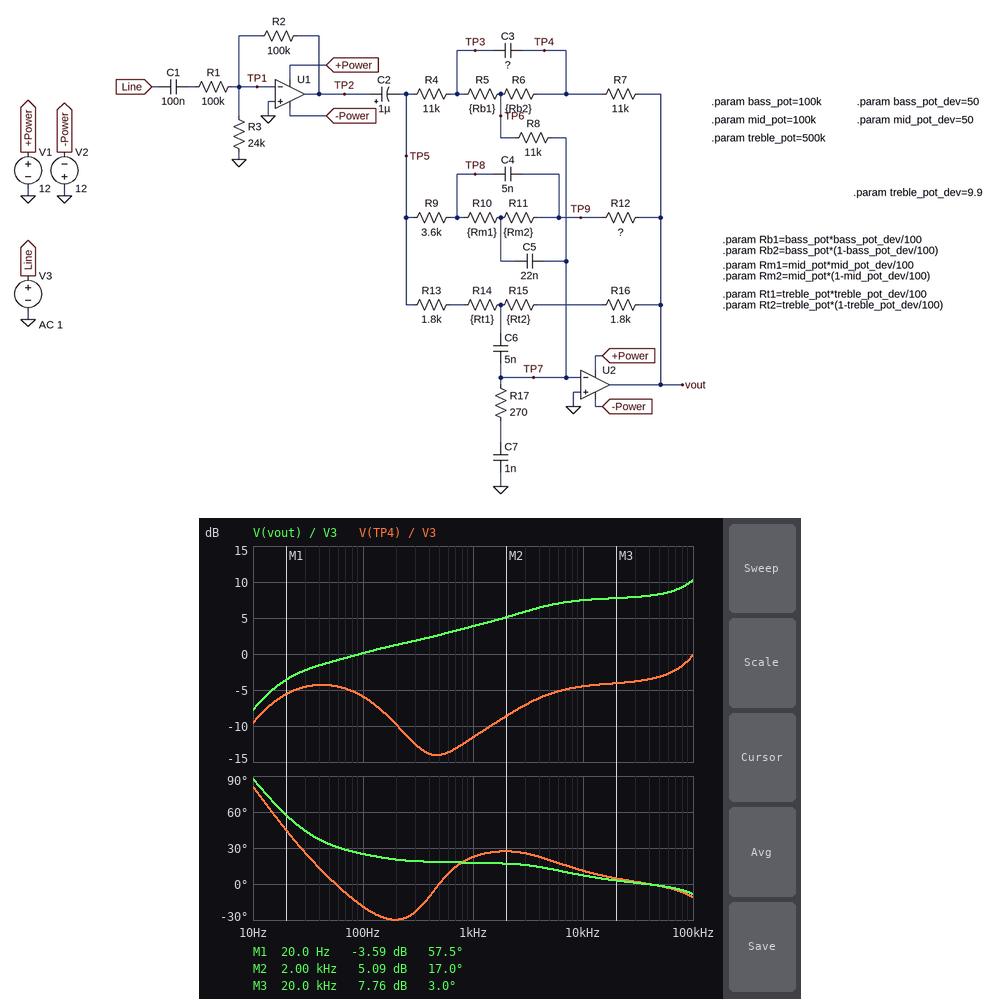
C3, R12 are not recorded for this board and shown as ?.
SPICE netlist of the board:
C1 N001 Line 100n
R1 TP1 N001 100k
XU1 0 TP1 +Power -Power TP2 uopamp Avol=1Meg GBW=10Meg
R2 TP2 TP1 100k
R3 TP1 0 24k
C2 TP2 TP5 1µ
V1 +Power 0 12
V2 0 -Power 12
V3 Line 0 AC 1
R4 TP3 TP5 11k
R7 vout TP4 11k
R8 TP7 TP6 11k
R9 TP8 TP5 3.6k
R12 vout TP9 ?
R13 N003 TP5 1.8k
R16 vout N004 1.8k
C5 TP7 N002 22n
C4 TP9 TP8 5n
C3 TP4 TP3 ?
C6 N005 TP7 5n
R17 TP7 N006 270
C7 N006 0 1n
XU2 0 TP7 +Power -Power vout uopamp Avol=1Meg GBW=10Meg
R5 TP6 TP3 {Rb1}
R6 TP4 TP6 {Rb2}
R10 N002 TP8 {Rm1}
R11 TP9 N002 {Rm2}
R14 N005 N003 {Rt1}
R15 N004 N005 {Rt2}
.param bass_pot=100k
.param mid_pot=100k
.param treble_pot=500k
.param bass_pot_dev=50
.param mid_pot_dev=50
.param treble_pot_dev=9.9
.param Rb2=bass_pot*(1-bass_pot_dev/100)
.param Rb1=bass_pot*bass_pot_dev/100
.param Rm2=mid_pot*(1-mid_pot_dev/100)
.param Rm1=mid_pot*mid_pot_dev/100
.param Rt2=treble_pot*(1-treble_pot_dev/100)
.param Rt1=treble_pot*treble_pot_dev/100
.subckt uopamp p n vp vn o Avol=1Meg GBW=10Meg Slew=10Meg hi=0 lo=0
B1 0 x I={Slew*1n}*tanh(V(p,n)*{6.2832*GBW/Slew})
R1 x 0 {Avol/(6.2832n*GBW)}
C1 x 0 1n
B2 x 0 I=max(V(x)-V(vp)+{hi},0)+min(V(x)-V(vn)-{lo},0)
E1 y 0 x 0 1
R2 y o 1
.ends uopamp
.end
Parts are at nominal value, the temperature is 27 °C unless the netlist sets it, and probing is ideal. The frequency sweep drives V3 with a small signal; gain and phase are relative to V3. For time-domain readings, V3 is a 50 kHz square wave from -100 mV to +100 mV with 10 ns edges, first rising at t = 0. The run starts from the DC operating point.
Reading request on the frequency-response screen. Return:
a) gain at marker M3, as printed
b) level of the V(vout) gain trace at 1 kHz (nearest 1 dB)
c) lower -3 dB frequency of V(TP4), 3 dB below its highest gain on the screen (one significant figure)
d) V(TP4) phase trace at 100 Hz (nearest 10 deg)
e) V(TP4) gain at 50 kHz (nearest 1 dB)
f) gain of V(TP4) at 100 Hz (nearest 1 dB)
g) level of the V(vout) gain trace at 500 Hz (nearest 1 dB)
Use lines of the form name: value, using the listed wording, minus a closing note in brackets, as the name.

gain at marker M3, as printed: 7.76 dB
level of the V(vout) gain trace at 1 kHz: 4 dB
lower -3 dB frequency of V(TP4), 3 dB below its highest gain on the screen: 50 kHz
V(TP4) phase trace at 100 Hz: -20 deg
V(TP4) gain at 50 kHz: -3 dB
gain of V(TP4) at 100 Hz: -6 dB
level of the V(vout) gain trace at 500 Hz: 3 dB
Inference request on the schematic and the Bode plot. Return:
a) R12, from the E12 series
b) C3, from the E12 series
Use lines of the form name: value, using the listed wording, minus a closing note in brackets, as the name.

R12, from the E12 series: 10 kΩ
C3, from the E12 series: 100 nF
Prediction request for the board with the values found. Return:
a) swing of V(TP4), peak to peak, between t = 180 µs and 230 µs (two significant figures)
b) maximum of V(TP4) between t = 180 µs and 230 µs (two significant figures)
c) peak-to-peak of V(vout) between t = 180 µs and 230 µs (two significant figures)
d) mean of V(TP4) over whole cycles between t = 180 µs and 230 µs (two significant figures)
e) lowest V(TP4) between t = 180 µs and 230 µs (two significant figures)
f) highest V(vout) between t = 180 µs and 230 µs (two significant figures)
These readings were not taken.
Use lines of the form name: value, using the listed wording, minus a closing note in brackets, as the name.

swing of V(TP4), peak to peak, between t = 180 µs and 230 µs: 350 mV
maximum of V(TP4) between t = 180 µs and 230 µs: 200 mV
peak-to-peak of V(vout) between t = 180 µs and 230 µs: 1.0 V
mean of V(TP4) over whole cycles between t = 180 µs and 230 µs: 25 mV
lowest V(TP4) between t = 180 µs and 230 µs: -150 mV
highest V(vout) between t = 180 µs and 230 µs: 640 mV
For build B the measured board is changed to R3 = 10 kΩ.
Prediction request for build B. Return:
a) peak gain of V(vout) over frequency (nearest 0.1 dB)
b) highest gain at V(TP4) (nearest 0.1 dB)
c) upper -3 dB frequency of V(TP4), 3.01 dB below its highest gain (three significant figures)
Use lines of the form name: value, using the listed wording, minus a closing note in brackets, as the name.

peak gain of V(vout) over frequency: 16.3 dB
highest gain at V(TP4): 8.6 dB
upper -3 dB frequency of V(TP4), 3.01 dB below its highest gain: 231 kHz
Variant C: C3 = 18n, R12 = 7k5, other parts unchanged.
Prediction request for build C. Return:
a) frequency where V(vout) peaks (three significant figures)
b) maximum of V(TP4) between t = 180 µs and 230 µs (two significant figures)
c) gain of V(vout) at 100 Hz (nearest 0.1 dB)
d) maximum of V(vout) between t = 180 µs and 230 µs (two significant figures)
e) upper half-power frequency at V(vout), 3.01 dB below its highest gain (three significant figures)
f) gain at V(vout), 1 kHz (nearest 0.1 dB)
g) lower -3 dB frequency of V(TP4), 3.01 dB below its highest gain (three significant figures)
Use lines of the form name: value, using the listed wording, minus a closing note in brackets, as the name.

frequency where V(vout) peaks: 194 kHz
maximum of V(TP4) between t = 180 µs and 230 µs: 210 mV
gain of V(vout) at 100 Hz: 0.4 dB
maximum of V(vout) between t = 180 µs and 230 µs: 570 mV
upper half-power frequency at V(vout), 3.01 dB below its highest gain: 232 kHz
gain at V(vout), 1 kHz: 3.5 dB
lower -3 dB frequency of V(TP4), 3.01 dB below its highest gain: 162 kHz
